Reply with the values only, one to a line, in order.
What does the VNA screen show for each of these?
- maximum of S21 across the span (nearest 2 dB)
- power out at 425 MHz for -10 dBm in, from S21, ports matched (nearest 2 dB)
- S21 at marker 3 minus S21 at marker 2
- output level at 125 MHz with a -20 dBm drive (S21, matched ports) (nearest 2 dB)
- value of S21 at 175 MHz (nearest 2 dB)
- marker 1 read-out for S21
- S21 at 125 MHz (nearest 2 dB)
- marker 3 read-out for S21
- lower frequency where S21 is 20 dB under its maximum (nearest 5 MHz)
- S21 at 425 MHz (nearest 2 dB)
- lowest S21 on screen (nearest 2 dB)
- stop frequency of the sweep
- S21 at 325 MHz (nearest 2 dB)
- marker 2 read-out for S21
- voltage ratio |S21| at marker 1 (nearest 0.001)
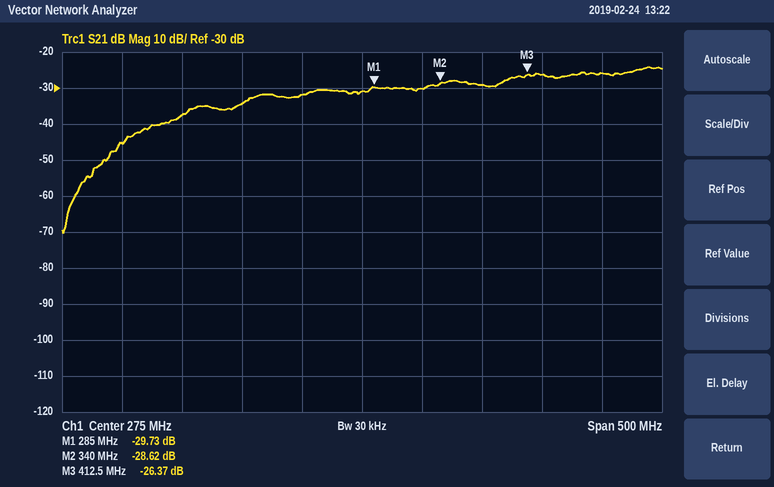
-24 dB
-36 dBm
2.25 dB
-58 dBm
-34 dB
-29.73 dB
-38 dB
-26.37 dB
80 MHz
-26 dB
-70 dB
525 MHz
-30 dB
-28.62 dB
0.033
